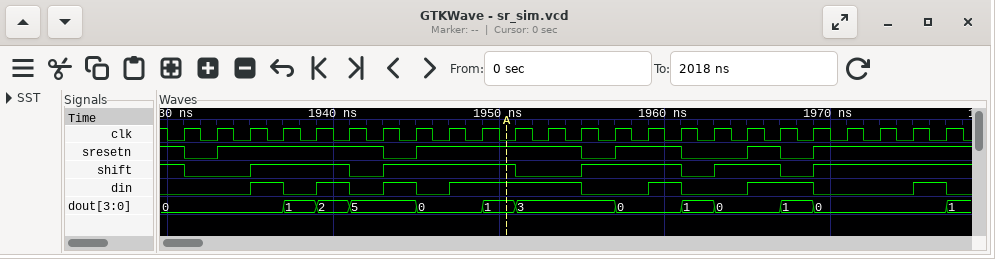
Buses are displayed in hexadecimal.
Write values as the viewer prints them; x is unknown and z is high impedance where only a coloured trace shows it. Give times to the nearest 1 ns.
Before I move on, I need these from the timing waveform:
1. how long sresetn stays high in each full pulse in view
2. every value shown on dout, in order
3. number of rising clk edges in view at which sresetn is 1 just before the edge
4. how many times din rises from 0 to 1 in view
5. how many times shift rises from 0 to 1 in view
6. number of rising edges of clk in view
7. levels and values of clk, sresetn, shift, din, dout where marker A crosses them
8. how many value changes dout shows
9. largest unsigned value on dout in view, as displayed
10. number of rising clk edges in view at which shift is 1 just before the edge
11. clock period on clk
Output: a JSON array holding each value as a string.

["10 ns, 10 ns, 4 ns, 2 ns", "0, 1, 2, 5, 0, 1, 3, 0, 1, 0, 1, 0, 1", "18", "7", "5", "24", "clk=0, sresetn=1, shift=1, din=1, dout=1", "12", "5", "17", "2 ns"]
